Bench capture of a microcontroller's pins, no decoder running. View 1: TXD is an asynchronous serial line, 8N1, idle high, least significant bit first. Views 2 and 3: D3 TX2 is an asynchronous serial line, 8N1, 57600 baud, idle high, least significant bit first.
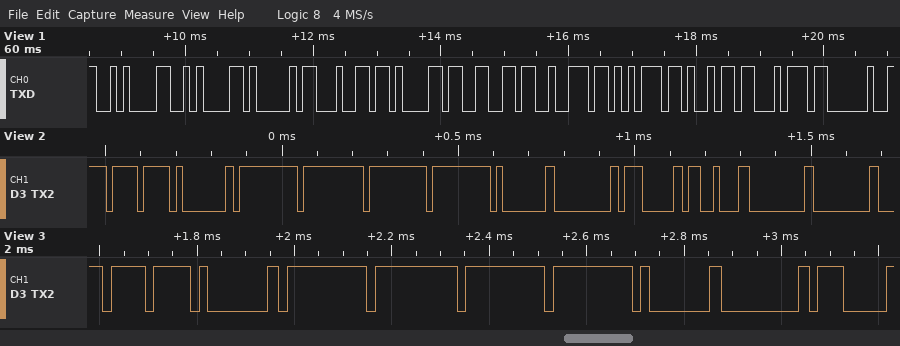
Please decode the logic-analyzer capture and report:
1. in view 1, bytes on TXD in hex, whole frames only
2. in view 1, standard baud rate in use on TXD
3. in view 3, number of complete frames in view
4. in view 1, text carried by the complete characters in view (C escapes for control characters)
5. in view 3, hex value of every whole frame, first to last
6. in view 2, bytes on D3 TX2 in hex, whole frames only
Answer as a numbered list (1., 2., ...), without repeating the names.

1. 0x0A 0x0A 0x41 0x64 0x61 0x66 0x72 0x75 0x69 0x74 0x20
2. 9600 baud
3. 9
4. "\n\nAdafruit "
5. 0xEF 0x01 0xFF 0xFF 0xFF 0xFF 0x01 0x00 0x07
6. 0xEF 0x01 0xFF 0xFF 0xFF 0xFF 0x01 0x00 0x07 0x13 0x00 0x00
